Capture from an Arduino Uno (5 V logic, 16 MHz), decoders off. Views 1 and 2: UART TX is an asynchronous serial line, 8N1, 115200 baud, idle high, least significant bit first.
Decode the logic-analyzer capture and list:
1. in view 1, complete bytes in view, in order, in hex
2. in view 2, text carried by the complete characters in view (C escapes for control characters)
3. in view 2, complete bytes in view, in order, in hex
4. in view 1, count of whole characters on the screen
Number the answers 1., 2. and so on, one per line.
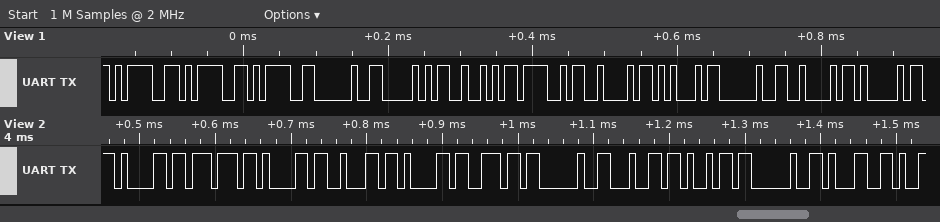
1. 3D 3D 3D 20 50 52 4F 42 45 20 42 41
2. "awaban di 1"
3. 61 77 61 62 61 6E 20 64 69 20 31
4. 12
